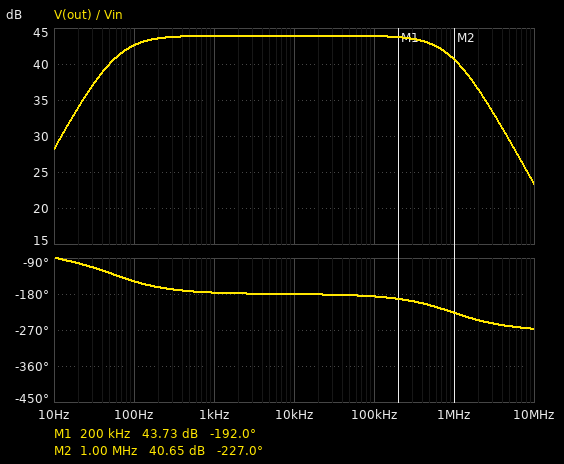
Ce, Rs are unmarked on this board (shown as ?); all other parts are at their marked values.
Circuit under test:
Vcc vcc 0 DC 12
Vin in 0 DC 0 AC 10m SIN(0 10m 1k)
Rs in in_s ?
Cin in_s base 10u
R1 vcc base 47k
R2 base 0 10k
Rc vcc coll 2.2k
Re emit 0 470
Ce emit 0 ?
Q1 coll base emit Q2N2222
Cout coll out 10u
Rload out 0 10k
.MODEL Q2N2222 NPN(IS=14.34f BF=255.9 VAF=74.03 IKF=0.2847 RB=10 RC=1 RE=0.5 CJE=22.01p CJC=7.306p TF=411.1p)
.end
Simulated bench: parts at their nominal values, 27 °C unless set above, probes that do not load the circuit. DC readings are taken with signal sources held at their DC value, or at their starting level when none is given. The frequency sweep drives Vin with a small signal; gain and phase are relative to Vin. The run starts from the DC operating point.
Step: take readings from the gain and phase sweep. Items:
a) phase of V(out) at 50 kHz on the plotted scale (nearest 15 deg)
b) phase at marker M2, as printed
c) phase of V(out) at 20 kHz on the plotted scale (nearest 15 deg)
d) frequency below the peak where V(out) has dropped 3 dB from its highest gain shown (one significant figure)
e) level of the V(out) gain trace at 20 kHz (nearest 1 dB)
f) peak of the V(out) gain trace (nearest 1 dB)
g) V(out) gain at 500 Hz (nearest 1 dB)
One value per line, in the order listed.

-180 deg
-227.0 deg
-180 deg
60 Hz
44 dB
44 dB
44 dB
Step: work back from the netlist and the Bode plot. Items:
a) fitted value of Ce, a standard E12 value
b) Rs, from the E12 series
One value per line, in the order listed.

270 µF
220 Ω
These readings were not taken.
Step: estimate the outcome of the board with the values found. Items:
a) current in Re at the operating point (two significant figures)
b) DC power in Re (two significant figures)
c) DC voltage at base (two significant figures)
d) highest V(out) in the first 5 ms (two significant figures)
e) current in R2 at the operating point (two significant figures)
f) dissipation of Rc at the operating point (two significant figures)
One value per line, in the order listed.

2.9 mA
3.8 mW
2.0 V
1.5 V
200 µA
18 mW
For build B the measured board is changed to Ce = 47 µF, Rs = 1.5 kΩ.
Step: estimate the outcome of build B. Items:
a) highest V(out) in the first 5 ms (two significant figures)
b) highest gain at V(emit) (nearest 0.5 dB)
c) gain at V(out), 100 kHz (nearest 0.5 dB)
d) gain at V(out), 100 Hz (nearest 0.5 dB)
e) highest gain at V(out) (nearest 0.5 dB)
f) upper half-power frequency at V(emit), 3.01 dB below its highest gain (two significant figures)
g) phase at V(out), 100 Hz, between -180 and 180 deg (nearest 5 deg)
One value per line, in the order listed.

990 mV
-2.0 dB
39.0 dB
32.0 dB
40.0 dB
230 Hz
-115 deg
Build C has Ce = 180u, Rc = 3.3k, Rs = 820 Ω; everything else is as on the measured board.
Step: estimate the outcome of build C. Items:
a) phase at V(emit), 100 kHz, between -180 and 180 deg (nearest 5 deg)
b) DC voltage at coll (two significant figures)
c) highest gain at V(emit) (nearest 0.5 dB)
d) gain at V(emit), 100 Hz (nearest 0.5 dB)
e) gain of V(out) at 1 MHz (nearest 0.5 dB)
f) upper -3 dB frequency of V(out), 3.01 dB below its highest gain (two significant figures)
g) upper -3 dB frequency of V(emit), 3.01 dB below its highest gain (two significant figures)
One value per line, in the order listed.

-120 deg
2.6 V
-2.0 dB
-6.5 dB
29.5 dB
180 kHz
74 Hz
